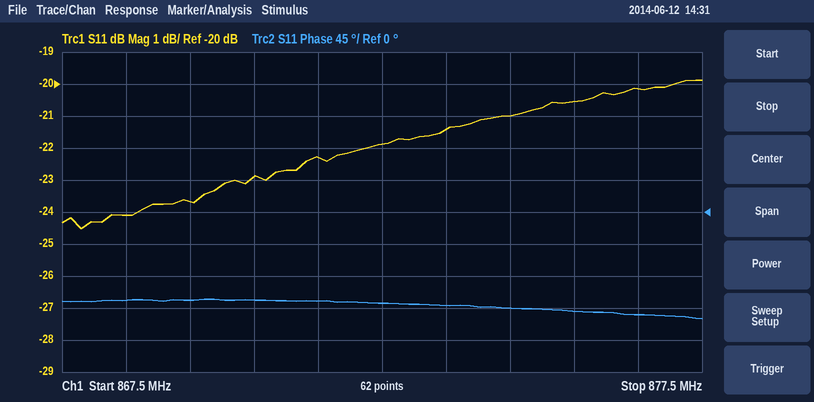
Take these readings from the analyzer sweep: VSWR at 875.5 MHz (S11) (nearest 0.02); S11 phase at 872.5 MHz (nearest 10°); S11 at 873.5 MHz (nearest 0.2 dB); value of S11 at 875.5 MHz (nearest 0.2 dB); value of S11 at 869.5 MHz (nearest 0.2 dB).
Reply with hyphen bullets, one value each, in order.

- 1.20
- -130°
- -21.4 dB
- -20.6 dB
- -23.6 dB
